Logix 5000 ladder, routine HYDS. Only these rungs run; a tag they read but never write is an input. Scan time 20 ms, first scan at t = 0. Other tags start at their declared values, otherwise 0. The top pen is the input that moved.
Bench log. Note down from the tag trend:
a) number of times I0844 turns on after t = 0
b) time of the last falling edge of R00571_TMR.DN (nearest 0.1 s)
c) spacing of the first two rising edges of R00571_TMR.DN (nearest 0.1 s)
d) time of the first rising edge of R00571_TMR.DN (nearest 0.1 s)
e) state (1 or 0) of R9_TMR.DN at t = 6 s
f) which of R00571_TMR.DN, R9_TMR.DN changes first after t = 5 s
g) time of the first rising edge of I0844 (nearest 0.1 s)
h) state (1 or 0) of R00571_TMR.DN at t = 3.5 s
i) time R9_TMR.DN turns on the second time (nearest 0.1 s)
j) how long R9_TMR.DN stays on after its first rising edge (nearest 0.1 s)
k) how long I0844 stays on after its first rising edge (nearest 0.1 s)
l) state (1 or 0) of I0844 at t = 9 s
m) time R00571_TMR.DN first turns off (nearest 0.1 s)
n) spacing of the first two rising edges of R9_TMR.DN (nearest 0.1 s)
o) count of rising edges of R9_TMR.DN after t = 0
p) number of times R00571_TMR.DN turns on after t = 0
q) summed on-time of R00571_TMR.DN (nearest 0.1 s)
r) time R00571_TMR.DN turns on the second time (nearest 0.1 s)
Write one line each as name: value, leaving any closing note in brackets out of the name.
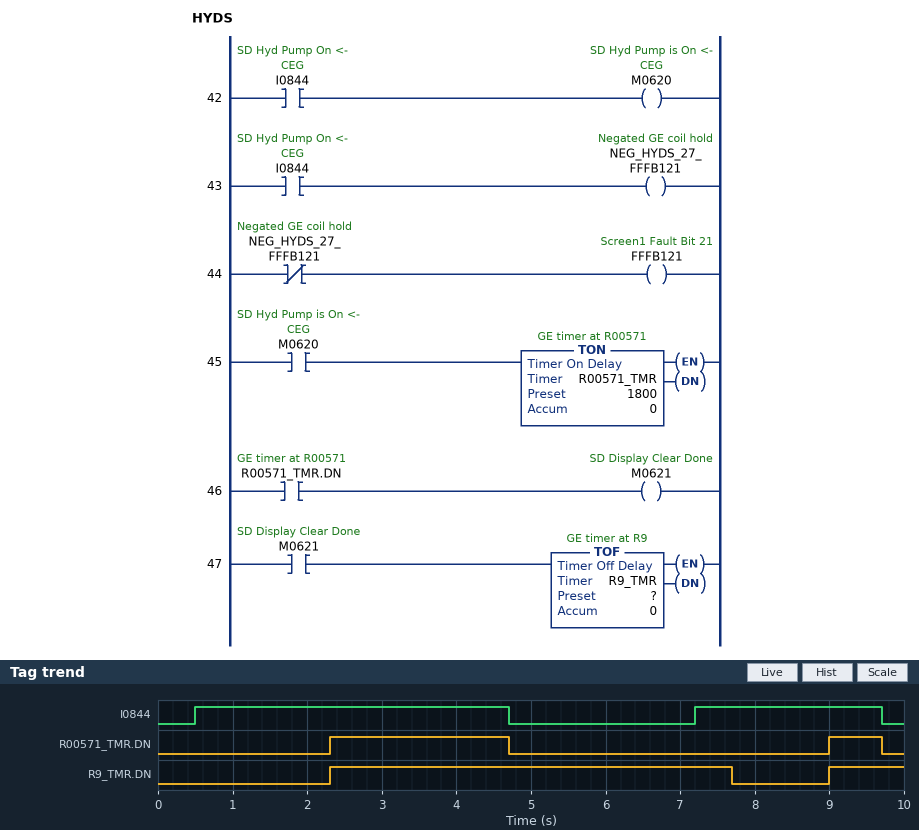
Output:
number of times I0844 turns on after t = 0: 2
time of the last falling edge of R00571_TMR.DN: 9.7 s
spacing of the first two rising edges of R00571_TMR.DN: 6.7 s
time of the first rising edge of R00571_TMR.DN: 2.3 s
state (1 or 0) of R9_TMR.DN at t = 6 s: 1
which of R00571_TMR.DN, R9_TMR.DN changes first after t = 5 s: R9_TMR.DN
time of the first rising edge of I0844: 0.5 s
state (1 or 0) of R00571_TMR.DN at t = 3.5 s: 1
time R9_TMR.DN turns on the second time: 9.0 s
how long R9_TMR.DN stays on after its first rising edge: 5.4 s
how long I0844 stays on after its first rising edge: 4.2 s
state (1 or 0) of I0844 at t = 9 s: 1
time R00571_TMR.DN first turns off: 4.7 s
spacing of the first two rising edges of R9_TMR.DN: 6.7 s
count of rising edges of R9_TMR.DN after t = 0: 2
number of times R00571_TMR.DN turns on after t = 0: 2
summed on-time of R00571_TMR.DN: 3.1 s
time R00571_TMR.DN turns on the second time: 9.0 s
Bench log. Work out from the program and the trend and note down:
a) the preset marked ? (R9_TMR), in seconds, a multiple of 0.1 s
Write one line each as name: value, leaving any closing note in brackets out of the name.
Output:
the preset marked ? (R9_TMR), in seconds, a multiple of 0.1 s: 3.0 s
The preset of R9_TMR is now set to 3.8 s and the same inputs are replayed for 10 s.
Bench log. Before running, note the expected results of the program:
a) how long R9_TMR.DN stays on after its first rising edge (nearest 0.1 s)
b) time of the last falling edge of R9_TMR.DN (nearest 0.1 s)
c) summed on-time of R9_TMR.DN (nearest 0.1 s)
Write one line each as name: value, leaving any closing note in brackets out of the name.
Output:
how long R9_TMR.DN stays on after its first rising edge: 6.2 s
time of the last falling edge of R9_TMR.DN: 8.5 s
summed on-time of R9_TMR.DN: 7.2 s
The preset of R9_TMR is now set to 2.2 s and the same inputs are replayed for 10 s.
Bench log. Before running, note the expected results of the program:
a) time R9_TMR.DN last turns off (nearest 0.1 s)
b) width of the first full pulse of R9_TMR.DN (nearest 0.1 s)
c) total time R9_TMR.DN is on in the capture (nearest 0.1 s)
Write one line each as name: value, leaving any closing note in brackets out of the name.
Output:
time R9_TMR.DN last turns off: 6.9 s
width of the first full pulse of R9_TMR.DN: 4.6 s
total time R9_TMR.DN is on in the capture: 5.6 s
